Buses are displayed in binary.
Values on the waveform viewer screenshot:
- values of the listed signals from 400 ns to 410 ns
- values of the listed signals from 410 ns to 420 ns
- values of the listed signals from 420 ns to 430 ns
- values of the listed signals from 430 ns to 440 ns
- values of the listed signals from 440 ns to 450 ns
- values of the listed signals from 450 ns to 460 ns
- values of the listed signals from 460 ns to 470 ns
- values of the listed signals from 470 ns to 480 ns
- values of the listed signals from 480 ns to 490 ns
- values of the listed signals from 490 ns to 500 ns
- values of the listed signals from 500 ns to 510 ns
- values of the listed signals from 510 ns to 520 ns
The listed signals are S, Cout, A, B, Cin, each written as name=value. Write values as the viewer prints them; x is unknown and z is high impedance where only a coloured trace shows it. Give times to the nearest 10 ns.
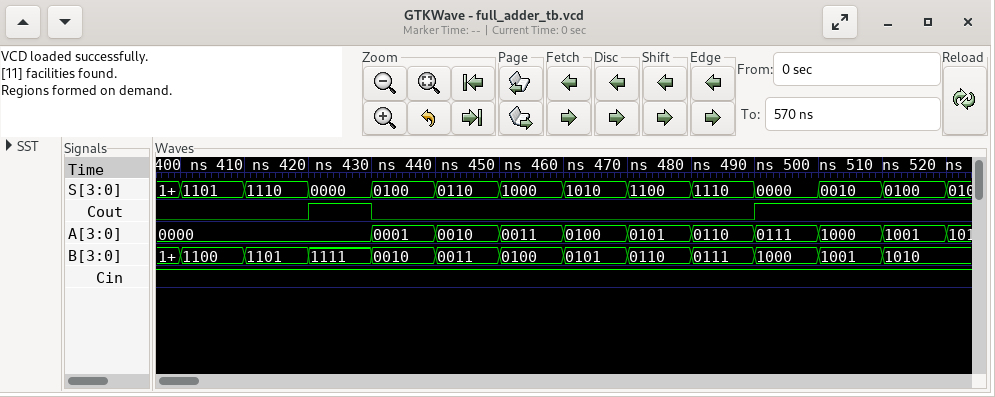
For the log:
S=1101, Cout=0, A=0000, B=1100, Cin=1
S=1110, Cout=0, A=0000, B=1101, Cin=1
S=0000, Cout=1, A=0000, B=1111, Cin=1
S=0100, Cout=0, A=0001, B=0010, Cin=1
S=0110, Cout=0, A=0010, B=0011, Cin=1
S=1000, Cout=0, A=0011, B=0100, Cin=1
S=1010, Cout=0, A=0100, B=0101, Cin=1
S=1100, Cout=0, A=0101, B=0110, Cin=1
S=1110, Cout=0, A=0110, B=0111, Cin=1
S=0000, Cout=1, A=0111, B=1000, Cin=1
S=0010, Cout=1, A=1000, B=1001, Cin=1
S=0100, Cout=1, A=1001, B=1010, Cin=1
